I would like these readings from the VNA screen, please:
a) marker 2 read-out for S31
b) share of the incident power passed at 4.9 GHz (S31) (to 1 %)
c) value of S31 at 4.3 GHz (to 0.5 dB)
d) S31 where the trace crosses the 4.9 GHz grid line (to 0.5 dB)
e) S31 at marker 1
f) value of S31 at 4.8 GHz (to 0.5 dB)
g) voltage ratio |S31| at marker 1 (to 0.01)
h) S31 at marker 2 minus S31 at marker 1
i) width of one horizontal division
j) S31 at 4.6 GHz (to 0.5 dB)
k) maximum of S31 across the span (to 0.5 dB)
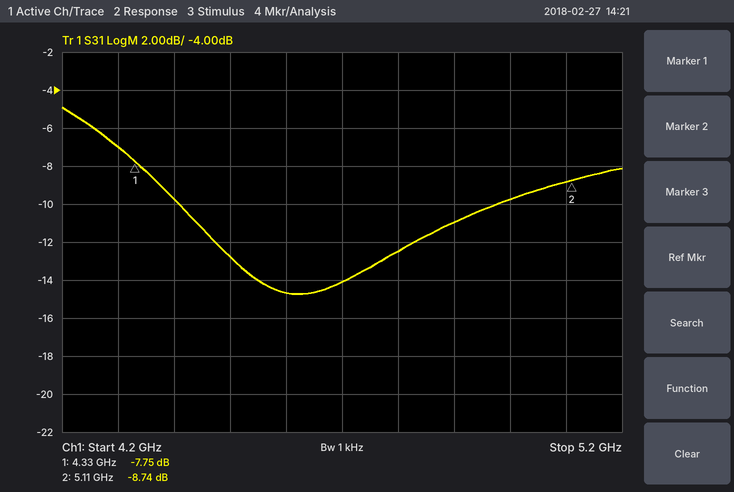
-8.74 dB
8 %
-7.0 dB
-11.0 dB
-7.75 dB
-12.5 dB
0.41
-0.99 dB
100 MHz
-14.5 dB
-5.0 dB
